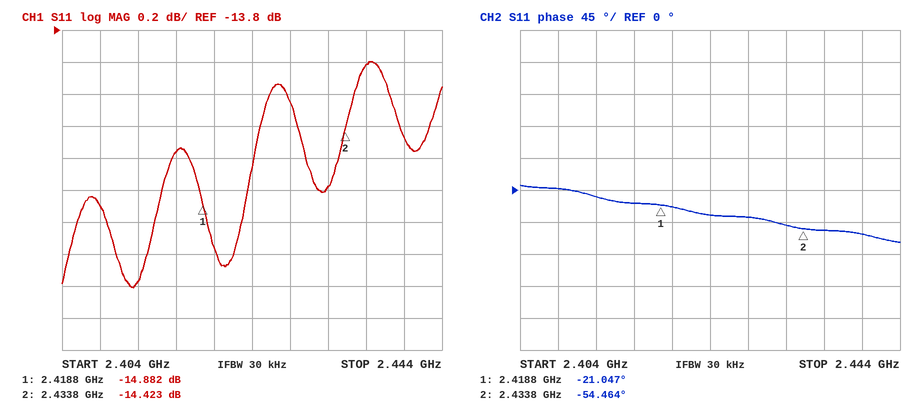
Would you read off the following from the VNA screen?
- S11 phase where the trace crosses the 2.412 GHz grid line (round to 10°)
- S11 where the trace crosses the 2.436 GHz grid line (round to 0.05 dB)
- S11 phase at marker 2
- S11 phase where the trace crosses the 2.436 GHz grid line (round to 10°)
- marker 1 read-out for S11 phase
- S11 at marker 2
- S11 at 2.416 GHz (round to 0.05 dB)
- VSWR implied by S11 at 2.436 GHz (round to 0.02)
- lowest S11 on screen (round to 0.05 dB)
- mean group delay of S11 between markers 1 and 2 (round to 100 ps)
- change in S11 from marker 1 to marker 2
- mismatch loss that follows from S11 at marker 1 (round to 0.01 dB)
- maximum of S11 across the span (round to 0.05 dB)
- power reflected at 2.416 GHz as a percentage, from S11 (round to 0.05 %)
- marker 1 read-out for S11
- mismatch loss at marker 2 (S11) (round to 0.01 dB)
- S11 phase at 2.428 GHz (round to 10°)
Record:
-10°
-14.00 dB
-54.464°
-60°
-21.047°
-14.423 dB
-14.55 dB
1.50
-15.40 dB
6.2 ns
0.459 dB
0.14 dB
-14.00 dB
3.50 %
-14.882 dB
0.16 dB
-40°
